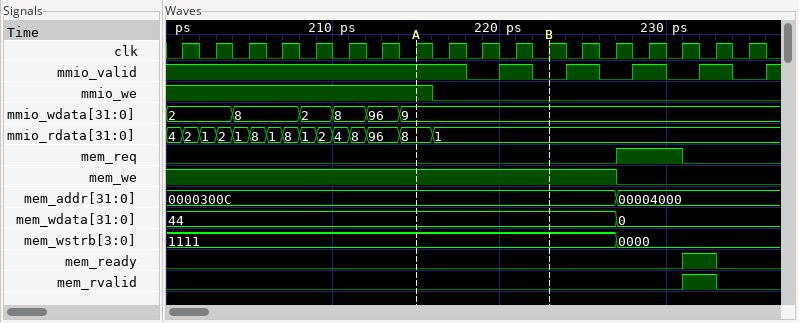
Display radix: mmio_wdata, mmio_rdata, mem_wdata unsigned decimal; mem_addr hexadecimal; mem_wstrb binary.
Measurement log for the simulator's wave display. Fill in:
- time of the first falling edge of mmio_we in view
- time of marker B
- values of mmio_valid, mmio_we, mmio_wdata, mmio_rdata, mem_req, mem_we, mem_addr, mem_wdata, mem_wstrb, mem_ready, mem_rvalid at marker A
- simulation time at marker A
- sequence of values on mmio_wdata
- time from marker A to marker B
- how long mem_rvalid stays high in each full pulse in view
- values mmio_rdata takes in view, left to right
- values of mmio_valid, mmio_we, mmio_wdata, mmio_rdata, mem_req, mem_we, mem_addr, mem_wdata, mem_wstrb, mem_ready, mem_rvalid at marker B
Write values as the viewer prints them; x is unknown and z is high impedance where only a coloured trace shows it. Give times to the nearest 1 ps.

216 ps
223 ps
mmio_valid=1, mmio_we=1, mmio_wdata=9, mmio_rdata=8, mem_req=0, mem_we=1, mem_addr=0000300C, mem_wdata=44, mem_wstrb=1111, mem_ready=0, mem_rvalid=0
215 ps
2, 8, 2, 8, 96, 9
8 ps
2 ps
4, 2, 1, 2, 1, 8, 1, 8, 1, 2, 4, 8, 96, 8, 1
mmio_valid=0, mmio_we=0, mmio_wdata=9, mmio_rdata=1, mem_req=0, mem_we=1, mem_addr=0000300C, mem_wdata=44, mem_wstrb=1111, mem_ready=0, mem_rvalid=0
